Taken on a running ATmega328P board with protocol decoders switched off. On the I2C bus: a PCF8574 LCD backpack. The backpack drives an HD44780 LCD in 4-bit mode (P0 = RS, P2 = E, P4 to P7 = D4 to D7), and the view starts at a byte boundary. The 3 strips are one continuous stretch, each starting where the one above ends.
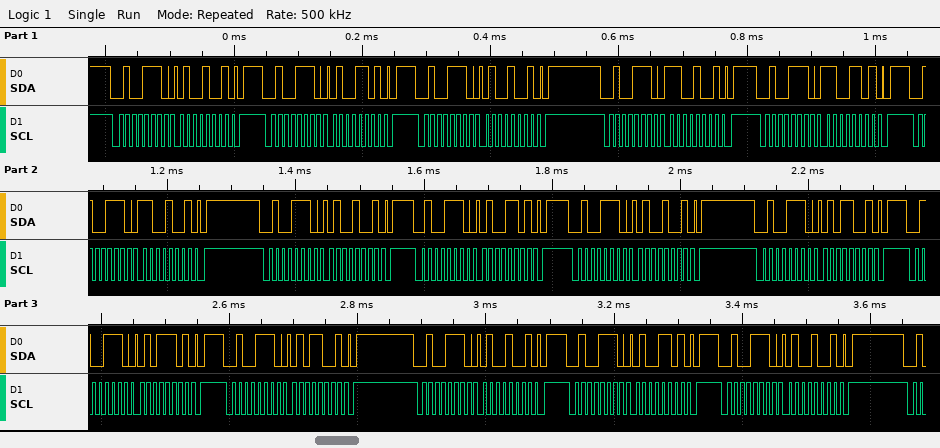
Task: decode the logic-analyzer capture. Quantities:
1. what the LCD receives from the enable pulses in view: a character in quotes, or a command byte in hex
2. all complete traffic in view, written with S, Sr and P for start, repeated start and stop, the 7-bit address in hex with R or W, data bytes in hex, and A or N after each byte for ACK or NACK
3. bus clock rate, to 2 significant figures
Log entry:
'L' 'E'
S 27W A 49 A P S 27W A 4D A P S 27W A 49 A P S 27W A C9 A P S 27W A CD A P S 27W A C9 A P S 27W A 49 A P S 27W A 4D A P S 27W A 49 A P S 27W A 59 A P S 27W A 5D A P S 27W A 59 A P S 27W A 49 A P S 27W A 4D A P S 27W A 49 A P
100 kHz
